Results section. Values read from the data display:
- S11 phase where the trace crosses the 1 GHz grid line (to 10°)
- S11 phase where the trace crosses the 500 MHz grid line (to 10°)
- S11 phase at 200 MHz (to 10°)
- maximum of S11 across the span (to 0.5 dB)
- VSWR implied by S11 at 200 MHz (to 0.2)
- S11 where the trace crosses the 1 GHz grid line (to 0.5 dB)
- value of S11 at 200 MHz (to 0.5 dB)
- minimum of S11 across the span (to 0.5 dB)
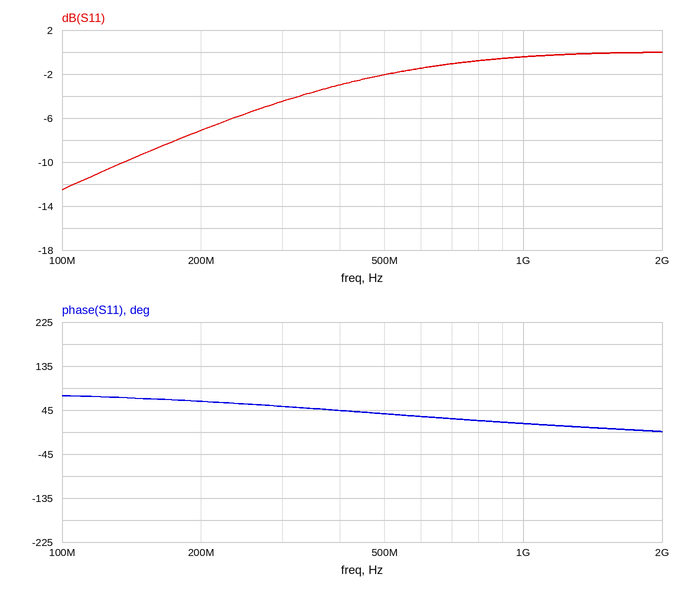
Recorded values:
20°
40°
60°
0.0 dB
2.6
-0.5 dB
-7.0 dB
-12.5 dB
